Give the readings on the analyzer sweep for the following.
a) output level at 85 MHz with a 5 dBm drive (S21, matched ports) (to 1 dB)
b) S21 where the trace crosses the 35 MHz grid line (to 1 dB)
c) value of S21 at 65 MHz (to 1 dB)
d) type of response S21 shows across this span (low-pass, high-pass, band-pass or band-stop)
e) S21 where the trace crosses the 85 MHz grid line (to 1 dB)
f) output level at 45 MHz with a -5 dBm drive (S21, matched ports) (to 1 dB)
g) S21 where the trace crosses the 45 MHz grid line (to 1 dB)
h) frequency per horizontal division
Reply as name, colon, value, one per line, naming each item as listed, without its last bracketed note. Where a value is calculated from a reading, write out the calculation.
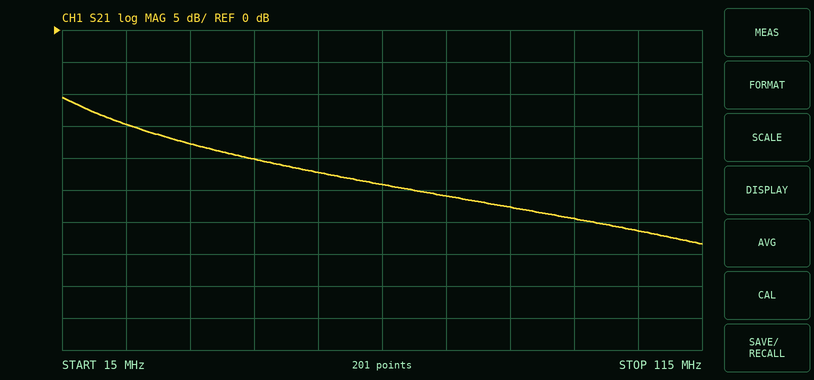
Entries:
output level at 85 MHz with a 5 dBm drive (S21, matched ports): 5 dBm + (-28 dB) = -23 dBm
S21 where the trace crosses the 35 MHz grid line: -18 dB
value of S21 at 65 MHz: -24 dB
type of response S21 shows across this span: low-pass
S21 where the trace crosses the 85 MHz grid line: -28 dB
output level at 45 MHz with a -5 dBm drive (S21, matched ports): -5 dBm + (-20 dB) = -25 dBm
S21 where the trace crosses the 45 MHz grid line: -20 dB
frequency per horizontal division: 10 MHz
